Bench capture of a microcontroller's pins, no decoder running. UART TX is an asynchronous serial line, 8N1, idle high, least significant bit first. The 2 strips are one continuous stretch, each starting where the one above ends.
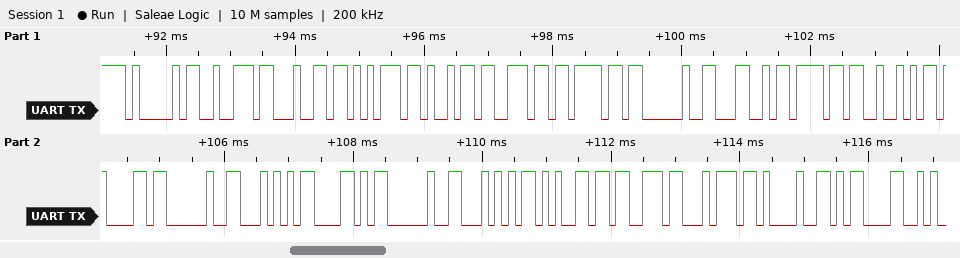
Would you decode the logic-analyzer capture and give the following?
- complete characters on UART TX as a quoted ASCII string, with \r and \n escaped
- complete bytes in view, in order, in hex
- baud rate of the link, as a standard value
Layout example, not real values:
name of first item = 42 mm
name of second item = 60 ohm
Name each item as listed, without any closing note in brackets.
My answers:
complete characters on UART TX as a quoted ASCII string, with \r and \n escaped = "Arduino LoRa TX Test!\r"
complete bytes in view, in order, in hex = 41 72 64 75 69 6E 6F 20 4C 6F 52 61 20 54 58 20 54 65 73 74 21 0D
baud rate of the link, as a standard value = 9600 baud
